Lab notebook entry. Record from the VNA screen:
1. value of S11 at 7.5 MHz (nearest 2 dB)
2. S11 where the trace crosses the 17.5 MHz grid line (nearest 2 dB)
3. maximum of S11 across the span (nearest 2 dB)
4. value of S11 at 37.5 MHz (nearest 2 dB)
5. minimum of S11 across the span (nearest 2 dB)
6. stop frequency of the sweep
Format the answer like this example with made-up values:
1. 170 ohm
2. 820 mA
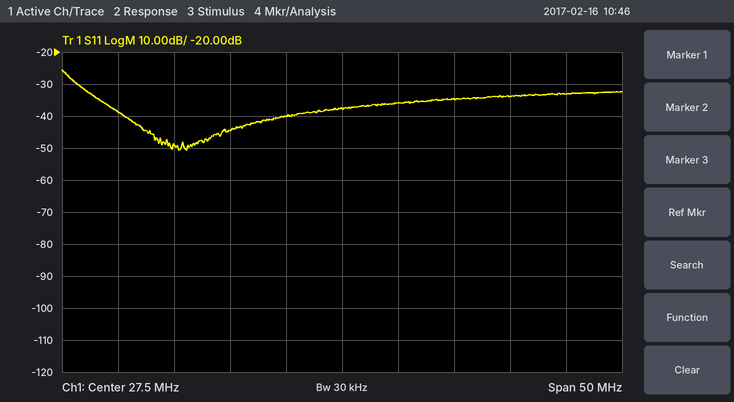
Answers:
1. -38 dB
2. -44 dB
3. -26 dB
4. -34 dB
5. -50 dB
6. 52.5 MHz
